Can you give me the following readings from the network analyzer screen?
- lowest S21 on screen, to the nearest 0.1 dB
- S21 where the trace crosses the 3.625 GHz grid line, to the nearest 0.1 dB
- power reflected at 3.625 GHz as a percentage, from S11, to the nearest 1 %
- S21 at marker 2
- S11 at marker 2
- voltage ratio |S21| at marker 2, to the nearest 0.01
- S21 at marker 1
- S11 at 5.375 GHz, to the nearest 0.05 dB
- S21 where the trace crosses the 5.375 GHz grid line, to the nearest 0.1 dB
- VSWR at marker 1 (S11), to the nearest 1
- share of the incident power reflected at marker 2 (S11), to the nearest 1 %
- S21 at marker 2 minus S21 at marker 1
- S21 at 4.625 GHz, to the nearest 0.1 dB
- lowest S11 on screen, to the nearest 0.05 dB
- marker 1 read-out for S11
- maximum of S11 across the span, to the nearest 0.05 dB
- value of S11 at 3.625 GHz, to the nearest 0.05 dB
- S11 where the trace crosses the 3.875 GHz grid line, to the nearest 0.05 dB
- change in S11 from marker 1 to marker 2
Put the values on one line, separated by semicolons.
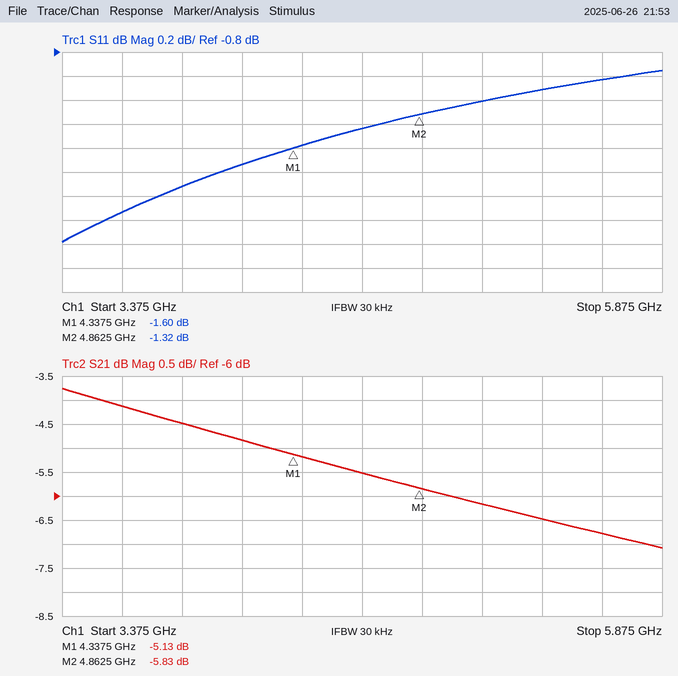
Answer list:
-7.1 dB; -4.1 dB; 61 %; -5.83 dB; -1.32 dB; 0.51; -5.13 dB; -1.10 dB; -6.5 dB; 11; 74 %; -0.70 dB; -5.5 dB; -2.40 dB; -1.60 dB; -0.95 dB; -2.15 dB; -1.90 dB; 0.28 dB
